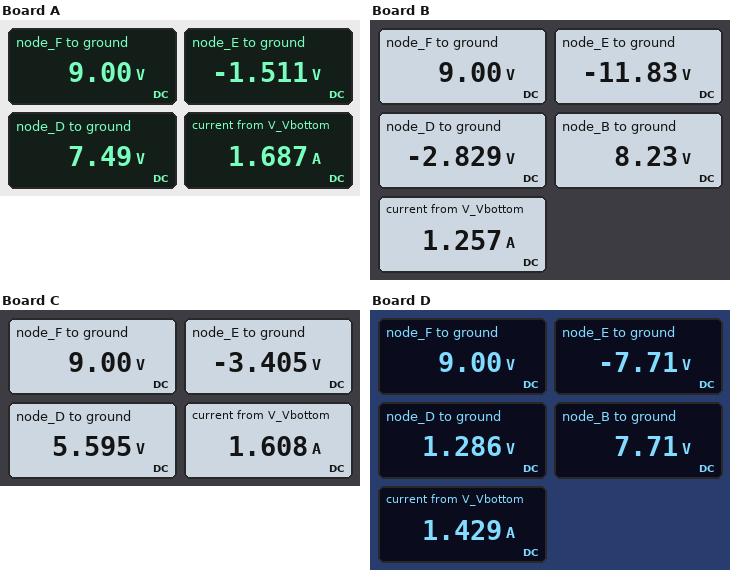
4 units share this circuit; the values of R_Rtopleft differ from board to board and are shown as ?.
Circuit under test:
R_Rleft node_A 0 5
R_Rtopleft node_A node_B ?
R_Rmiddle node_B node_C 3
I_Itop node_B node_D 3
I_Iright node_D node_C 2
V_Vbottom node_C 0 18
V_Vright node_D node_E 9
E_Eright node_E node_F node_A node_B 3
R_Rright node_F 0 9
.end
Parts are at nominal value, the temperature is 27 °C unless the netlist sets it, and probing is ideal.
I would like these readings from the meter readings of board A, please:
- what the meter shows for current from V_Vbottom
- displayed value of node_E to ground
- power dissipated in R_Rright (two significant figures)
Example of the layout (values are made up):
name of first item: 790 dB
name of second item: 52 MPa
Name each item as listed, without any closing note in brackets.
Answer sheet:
what the meter shows for current from V_Vbottom: 1.687 A
displayed value of node_E to ground: -1.511 V
power dissipated in R_Rright: 9.0 W
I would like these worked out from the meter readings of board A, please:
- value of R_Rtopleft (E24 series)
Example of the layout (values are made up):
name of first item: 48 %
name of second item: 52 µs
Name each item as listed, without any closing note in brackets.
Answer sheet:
value of R_Rtopleft: 5.1 Ω
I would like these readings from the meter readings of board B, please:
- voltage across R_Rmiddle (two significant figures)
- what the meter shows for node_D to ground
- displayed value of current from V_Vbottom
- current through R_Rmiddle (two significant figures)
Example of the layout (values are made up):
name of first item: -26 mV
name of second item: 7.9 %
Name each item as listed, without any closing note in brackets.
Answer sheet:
voltage across R_Rmiddle: 9.8 V
what the meter shows for node_D to ground: -2.829 V
displayed value of current from V_Vbottom: 1.257 A
current through R_Rmiddle: 3.3 A
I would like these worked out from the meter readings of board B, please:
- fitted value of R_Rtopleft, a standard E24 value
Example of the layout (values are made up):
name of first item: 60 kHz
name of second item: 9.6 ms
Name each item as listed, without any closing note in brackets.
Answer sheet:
fitted value of R_Rtopleft, a standard E24 value: 27 Ω
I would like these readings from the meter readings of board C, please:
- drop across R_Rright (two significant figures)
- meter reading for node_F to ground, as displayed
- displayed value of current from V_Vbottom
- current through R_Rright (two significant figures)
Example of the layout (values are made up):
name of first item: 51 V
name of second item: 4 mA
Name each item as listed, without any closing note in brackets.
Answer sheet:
drop across R_Rright: 9.0 V
meter reading for node_F to ground, as displayed: 9.00 V
displayed value of current from V_Vbottom: 1.608 A
current through R_Rright: 1.0 A
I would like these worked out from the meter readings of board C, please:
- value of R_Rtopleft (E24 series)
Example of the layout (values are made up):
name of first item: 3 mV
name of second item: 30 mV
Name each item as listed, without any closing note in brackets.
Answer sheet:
value of R_Rtopleft: 6.8 Ω
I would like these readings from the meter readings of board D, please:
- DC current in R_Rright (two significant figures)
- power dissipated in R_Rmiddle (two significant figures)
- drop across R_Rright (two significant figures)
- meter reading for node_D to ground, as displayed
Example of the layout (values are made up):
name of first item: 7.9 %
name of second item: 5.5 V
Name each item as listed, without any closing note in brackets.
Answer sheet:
DC current in R_Rright: 1.0 A
power dissipated in R_Rmiddle: 35 W
drop across R_Rright: 9.0 V
meter reading for node_D to ground, as displayed: 1.286 V
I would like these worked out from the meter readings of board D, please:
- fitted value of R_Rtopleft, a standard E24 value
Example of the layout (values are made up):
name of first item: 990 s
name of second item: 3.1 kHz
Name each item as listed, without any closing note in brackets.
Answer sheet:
fitted value of R_Rtopleft, a standard E24 value: 13 Ω
